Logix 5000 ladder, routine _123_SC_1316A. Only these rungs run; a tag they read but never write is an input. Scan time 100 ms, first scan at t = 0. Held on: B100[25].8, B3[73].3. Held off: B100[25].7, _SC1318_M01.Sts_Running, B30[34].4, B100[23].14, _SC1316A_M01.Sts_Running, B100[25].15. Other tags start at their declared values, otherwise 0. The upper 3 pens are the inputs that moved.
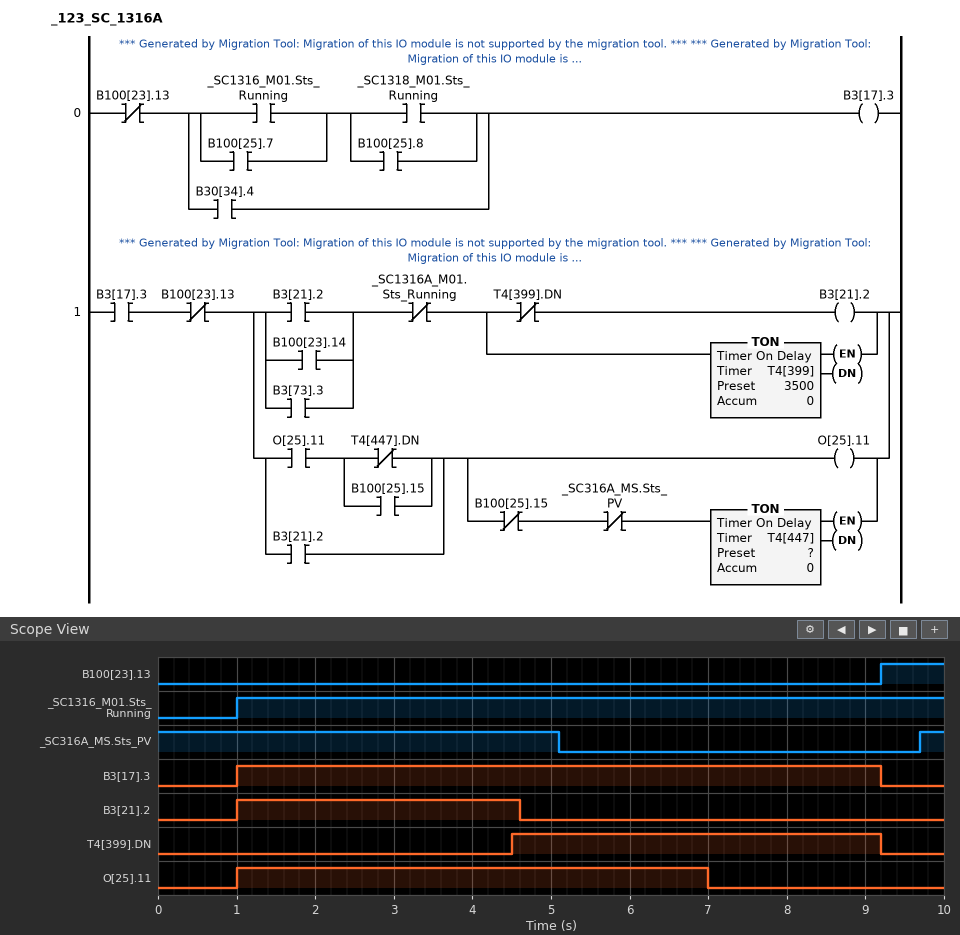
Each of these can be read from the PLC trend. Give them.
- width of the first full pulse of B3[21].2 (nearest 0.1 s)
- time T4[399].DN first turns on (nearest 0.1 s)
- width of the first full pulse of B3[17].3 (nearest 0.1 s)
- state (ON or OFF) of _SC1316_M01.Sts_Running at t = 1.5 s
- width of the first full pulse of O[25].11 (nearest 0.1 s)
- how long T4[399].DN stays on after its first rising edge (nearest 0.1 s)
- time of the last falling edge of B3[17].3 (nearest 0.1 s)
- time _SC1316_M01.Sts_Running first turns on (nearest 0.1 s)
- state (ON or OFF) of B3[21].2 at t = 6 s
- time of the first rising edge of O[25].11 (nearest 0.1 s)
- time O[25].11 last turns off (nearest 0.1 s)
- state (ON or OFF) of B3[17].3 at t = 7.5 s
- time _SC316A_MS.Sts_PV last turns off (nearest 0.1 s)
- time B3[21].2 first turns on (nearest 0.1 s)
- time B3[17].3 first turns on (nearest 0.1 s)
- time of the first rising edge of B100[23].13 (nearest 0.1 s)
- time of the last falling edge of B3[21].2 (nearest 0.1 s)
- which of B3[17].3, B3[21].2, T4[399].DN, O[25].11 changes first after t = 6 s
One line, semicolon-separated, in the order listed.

3.6 s; 4.5 s; 8.2 s; ON; 6.0 s; 4.7 s; 9.2 s; 1.0 s; OFF; 1.0 s; 7.0 s; ON; 5.1 s; 1.0 s; 1.0 s; 9.2 s; 4.6 s; O[25].11
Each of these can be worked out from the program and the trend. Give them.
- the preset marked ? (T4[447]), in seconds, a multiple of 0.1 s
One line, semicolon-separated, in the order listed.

1.8 s
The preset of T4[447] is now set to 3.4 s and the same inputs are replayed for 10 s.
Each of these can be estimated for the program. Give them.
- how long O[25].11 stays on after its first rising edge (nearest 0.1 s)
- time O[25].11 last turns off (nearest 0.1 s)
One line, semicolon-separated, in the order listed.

7.6 s; 8.6 s
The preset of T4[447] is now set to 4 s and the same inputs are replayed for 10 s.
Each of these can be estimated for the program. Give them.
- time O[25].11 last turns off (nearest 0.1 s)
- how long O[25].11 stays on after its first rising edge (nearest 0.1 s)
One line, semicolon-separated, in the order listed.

9.2 s; 8.2 s
